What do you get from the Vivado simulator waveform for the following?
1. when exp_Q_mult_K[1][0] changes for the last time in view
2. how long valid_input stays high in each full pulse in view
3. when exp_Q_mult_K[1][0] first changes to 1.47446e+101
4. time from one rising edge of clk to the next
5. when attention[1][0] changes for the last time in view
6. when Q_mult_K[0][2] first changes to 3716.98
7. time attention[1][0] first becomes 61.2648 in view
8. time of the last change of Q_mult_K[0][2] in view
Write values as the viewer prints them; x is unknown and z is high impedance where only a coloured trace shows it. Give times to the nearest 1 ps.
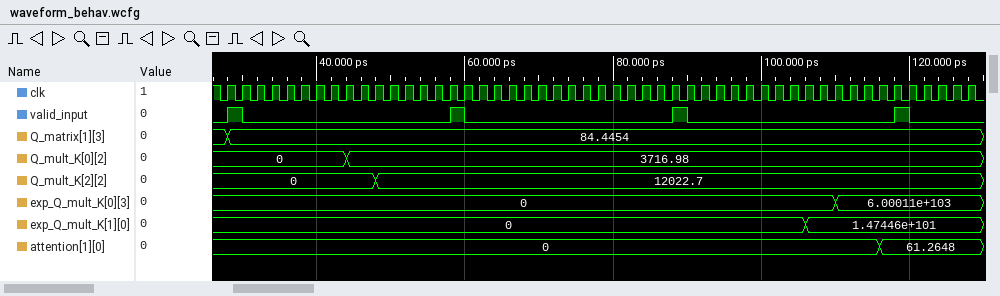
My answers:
106 ps
2 ps, 2 ps, 2 ps, 2 ps
106 ps
2 ps
116 ps
44 ps
116 ps
44 ps
